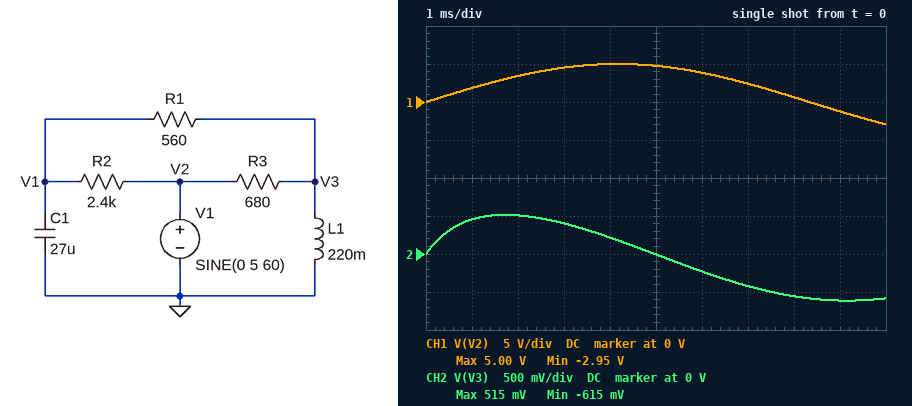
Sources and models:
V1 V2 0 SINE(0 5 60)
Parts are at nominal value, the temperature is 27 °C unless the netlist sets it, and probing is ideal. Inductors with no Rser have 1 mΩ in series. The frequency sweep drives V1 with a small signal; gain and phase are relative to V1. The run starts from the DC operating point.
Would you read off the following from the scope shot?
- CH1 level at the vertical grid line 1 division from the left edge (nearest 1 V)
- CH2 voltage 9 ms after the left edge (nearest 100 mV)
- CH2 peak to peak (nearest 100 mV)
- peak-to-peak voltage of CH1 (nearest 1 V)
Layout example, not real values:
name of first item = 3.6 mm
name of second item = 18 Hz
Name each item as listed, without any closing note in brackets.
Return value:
CH1 level at the vertical grid line 1 division from the left edge = 2 V
CH2 voltage 9 ms after the left edge = -600 mV
CH2 peak to peak = 1.1 V
peak-to-peak voltage of CH1 = 8 V
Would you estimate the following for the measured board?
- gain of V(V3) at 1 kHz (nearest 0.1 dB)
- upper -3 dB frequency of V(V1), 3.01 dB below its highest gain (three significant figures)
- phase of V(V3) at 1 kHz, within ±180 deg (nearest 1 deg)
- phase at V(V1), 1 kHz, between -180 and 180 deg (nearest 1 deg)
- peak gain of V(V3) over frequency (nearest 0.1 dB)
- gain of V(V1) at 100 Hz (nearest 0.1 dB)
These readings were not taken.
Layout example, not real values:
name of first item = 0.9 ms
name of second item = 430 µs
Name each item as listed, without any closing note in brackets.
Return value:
gain of V(V3) at 1 kHz = -7.1 dB
upper -3 dB frequency of V(V1), 3.01 dB below its highest gain = 13.7 Hz
phase of V(V3) at 1 kHz, within ±180 deg = 12 deg
phase at V(V1), 1 kHz, between -180 and 180 deg = -81 deg
peak gain of V(V3) over frequency = -6.9 dB
gain of V(V1) at 100 Hz = -28.5 dB
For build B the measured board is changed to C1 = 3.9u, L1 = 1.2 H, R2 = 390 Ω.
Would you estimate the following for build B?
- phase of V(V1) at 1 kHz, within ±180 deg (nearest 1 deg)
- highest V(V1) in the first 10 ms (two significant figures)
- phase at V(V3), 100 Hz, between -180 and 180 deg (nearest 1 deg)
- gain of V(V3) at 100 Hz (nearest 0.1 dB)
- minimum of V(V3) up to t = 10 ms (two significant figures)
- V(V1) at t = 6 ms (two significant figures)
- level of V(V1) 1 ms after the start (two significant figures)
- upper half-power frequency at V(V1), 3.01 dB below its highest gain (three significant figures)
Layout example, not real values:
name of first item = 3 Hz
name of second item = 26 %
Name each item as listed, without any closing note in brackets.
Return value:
phase of V(V1) at 1 kHz, within ±180 deg = -82 deg
highest V(V1) in the first 10 ms = 3.7 V
phase at V(V3), 100 Hz, between -180 and 180 deg = 9 deg
gain of V(V3) at 100 Hz = -1.9 dB
minimum of V(V3) up to t = 10 ms = -3.5 V
V(V1) at t = 6 ms = 3.3 V
level of V(V1) 1 ms after the start = 600 mV
upper half-power frequency at V(V1), 3.01 dB below its highest gain = 194 Hz
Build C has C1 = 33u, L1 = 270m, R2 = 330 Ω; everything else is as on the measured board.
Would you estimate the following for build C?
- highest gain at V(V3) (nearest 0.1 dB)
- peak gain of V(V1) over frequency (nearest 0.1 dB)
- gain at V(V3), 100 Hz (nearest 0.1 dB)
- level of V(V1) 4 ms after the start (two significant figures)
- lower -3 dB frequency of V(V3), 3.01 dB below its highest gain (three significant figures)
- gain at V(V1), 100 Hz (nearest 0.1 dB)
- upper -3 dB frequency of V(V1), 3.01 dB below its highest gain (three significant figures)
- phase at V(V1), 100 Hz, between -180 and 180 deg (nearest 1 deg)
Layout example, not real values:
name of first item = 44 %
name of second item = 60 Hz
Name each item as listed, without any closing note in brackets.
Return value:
highest gain at V(V3) = -6.9 dB
peak gain of V(V1) over frequency = -4.0 dB
gain at V(V3), 100 Hz = -12.6 dB
level of V(V1) 4 ms after the start = 1.0 V
lower -3 dB frequency of V(V3), 3.01 dB below its highest gain = 169 Hz
gain at V(V1), 100 Hz = -16.2 dB
upper -3 dB frequency of V(V1), 3.01 dB below its highest gain = 24.2 Hz
phase at V(V1), 100 Hz, between -180 and 180 deg = -71 deg
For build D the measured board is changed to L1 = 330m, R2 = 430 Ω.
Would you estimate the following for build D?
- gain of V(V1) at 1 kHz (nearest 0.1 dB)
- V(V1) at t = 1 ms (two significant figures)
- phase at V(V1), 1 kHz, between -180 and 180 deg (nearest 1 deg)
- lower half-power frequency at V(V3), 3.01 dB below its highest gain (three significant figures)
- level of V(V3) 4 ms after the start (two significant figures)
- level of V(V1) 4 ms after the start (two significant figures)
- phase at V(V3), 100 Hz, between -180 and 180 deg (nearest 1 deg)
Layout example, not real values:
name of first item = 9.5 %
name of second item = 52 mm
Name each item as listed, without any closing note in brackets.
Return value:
gain of V(V1) at 1 kHz = -34.7 dB
V(V1) at t = 1 ms = 97 mV
phase at V(V1), 1 kHz, between -180 and 180 deg = -87 deg
lower half-power frequency at V(V3), 3.01 dB below its highest gain = 134 Hz
level of V(V3) 4 ms after the start = 530 mV
level of V(V1) 4 ms after the start = 990 mV
phase at V(V3), 100 Hz, between -180 and 180 deg = 47 deg
